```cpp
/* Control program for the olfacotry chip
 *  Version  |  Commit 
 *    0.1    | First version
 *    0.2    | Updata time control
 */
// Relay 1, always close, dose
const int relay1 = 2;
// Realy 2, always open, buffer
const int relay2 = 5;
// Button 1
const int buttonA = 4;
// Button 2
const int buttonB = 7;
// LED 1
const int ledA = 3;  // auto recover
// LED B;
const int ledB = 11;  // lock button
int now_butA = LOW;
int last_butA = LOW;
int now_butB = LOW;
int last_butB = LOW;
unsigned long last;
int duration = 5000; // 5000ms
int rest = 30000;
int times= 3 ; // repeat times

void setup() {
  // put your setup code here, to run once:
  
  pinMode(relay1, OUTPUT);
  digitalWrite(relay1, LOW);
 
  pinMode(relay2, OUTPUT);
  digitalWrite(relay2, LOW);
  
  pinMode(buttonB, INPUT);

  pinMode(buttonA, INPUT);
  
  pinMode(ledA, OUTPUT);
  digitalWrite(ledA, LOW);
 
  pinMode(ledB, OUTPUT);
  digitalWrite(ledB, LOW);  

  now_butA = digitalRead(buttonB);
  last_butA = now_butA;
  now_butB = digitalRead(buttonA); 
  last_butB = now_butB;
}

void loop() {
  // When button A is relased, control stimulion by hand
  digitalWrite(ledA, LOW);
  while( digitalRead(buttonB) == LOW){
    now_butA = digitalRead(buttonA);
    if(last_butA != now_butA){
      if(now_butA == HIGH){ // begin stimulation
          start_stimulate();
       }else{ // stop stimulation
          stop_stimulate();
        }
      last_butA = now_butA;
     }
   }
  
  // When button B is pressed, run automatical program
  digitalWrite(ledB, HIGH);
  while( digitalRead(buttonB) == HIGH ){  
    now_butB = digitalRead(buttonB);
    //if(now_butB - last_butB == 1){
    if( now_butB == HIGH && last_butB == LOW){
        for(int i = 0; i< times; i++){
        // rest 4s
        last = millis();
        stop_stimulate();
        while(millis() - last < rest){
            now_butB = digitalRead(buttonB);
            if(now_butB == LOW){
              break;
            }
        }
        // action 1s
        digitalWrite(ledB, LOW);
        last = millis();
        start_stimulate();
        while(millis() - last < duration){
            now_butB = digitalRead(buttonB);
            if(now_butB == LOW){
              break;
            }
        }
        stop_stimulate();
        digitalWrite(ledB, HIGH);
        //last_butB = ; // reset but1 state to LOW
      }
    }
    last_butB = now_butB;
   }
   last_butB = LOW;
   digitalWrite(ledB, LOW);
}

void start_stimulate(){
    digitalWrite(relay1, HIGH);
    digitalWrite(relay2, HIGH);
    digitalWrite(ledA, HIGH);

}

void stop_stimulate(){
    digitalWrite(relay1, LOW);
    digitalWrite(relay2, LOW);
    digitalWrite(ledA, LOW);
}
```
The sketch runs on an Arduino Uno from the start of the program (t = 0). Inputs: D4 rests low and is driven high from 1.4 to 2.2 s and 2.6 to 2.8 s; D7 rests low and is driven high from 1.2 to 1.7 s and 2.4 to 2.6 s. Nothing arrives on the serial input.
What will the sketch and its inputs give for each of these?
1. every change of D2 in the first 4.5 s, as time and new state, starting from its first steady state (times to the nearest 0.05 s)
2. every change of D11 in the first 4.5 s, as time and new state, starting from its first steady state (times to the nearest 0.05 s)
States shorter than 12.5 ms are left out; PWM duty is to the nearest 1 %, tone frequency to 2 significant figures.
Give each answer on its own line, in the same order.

0 s low; 1.7 s high; 2.2 s low; 2.6 s high; 2.8 s low
0 s low; 1.2 s high; 1.7 s low; 2.4 s high; 2.6 s low
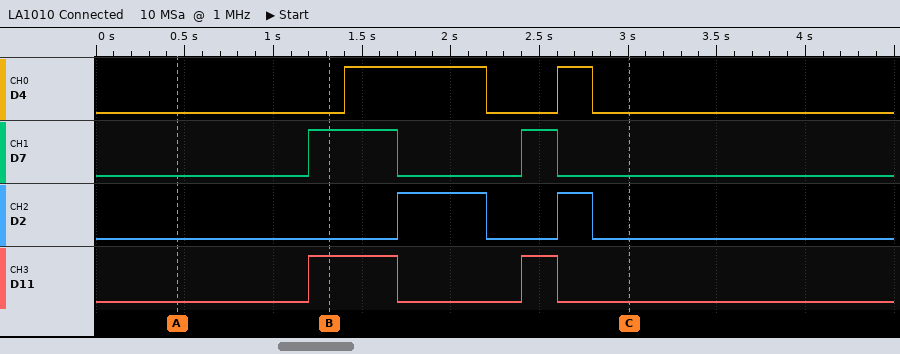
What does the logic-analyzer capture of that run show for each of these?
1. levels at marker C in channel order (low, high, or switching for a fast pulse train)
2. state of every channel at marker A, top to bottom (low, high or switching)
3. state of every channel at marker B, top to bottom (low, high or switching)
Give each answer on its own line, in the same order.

D4 low, D7 low, D2 low, D11 low
D4 low, D7 low, D2 low, D11 low
D4 low, D7 high, D2 low, D11 high
